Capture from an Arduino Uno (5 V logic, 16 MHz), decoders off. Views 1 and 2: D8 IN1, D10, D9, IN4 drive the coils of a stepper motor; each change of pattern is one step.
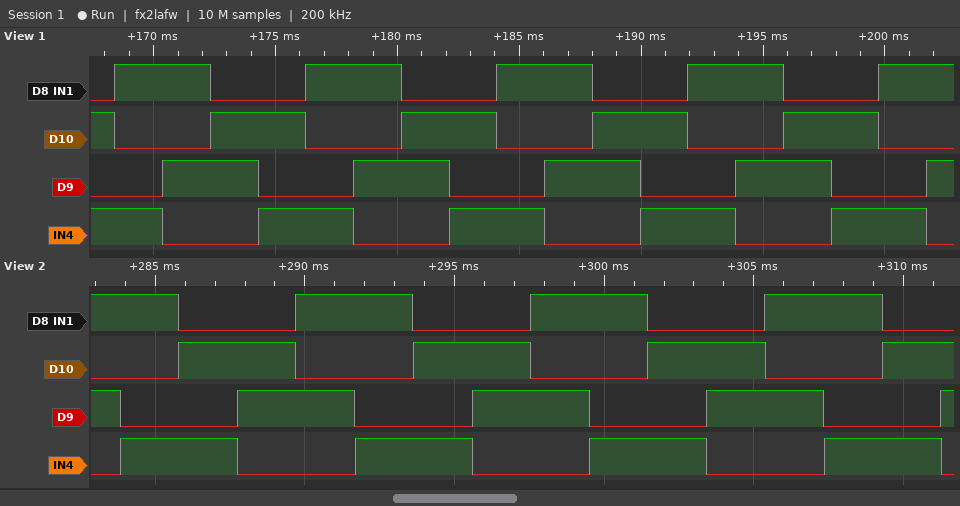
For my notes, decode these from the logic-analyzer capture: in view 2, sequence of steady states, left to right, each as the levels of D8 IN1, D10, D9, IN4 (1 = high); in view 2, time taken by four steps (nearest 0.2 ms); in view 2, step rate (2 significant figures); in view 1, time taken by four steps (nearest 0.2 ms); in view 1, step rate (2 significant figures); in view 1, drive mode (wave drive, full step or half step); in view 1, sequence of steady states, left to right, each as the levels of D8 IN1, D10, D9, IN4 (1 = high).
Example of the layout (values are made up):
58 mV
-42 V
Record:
1010 1001 0101 0110 1010 1001 0101 0110 1010 1001 0101 0110 1010 1001 0101 0110
7.8 ms
510 steps/s
7.8 ms
510 steps/s
full step
0101 1001 1010 0110 0101 1001 1010 0110 0101 1001 1010 0110 0101 1001 1010 0110 0101 1001 1010
